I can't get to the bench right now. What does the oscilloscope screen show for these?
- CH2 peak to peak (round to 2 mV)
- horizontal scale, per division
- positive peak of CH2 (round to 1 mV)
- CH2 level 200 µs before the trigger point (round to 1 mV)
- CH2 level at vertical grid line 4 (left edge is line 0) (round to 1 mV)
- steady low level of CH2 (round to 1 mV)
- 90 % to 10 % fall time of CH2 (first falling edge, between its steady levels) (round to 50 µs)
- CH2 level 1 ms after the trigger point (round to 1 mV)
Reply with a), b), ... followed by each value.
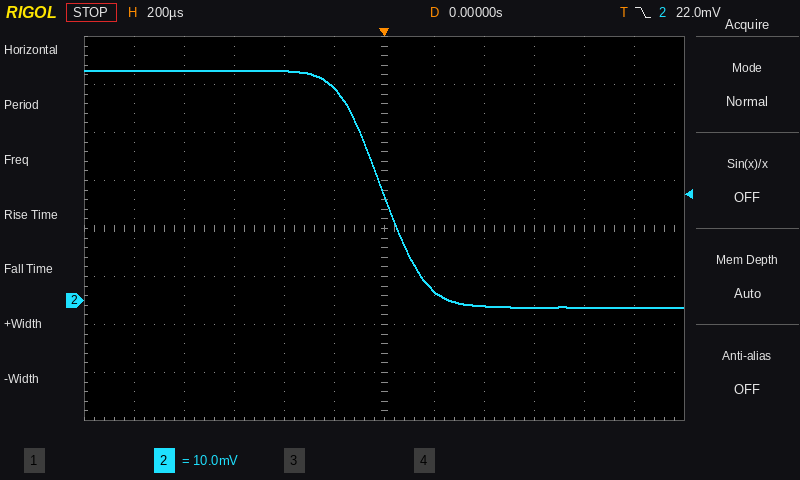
a) 50 mV
b) 200 µs
c) 48 mV
d) 44 mV
e) 48 mV
f) -1 mV
g) 350 µs
h) -1 mV
